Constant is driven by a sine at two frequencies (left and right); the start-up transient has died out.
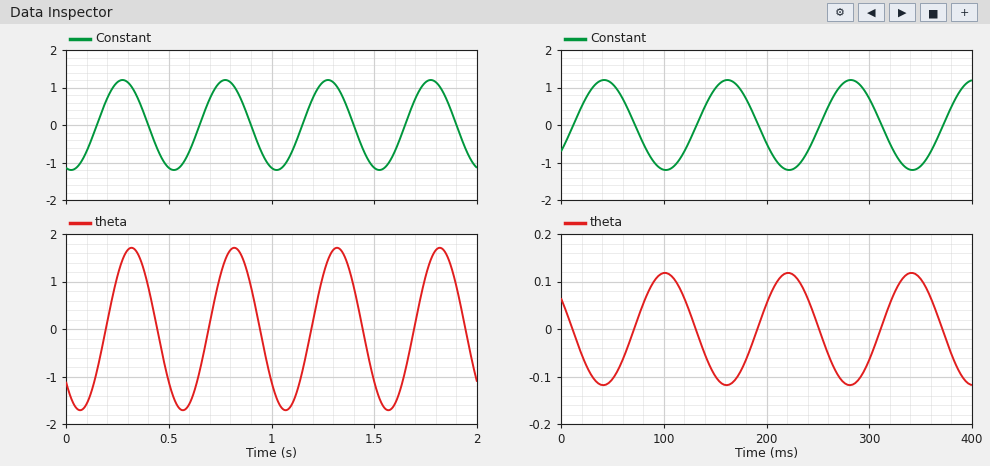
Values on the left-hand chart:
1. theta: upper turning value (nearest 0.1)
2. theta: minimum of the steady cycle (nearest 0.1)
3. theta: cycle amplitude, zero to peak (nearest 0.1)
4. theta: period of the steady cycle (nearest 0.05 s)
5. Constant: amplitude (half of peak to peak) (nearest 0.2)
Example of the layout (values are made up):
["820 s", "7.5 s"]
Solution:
["1.7", "-1.7", "1.7", "0.50 s", "1.2"]
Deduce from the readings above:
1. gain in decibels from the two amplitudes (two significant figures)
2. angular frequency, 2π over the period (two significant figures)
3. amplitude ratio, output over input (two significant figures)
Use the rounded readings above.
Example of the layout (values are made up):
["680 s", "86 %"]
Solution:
["3.0 dB", "13 rad/s", "1.4"]
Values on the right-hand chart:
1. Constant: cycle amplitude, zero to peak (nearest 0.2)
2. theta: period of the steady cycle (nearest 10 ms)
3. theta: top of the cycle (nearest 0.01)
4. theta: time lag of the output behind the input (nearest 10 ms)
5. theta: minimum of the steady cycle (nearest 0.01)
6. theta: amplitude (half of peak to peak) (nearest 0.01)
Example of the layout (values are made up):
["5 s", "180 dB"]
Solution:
["1.2", "120 ms", "0.12", "60 ms", "-0.12", "0.12"]
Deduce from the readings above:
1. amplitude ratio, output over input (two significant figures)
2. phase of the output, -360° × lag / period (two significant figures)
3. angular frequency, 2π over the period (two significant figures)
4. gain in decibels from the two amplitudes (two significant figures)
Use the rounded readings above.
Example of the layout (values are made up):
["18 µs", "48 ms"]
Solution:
["0.10", "-180°", "0.052 rad/ms", "-20 dB"]
